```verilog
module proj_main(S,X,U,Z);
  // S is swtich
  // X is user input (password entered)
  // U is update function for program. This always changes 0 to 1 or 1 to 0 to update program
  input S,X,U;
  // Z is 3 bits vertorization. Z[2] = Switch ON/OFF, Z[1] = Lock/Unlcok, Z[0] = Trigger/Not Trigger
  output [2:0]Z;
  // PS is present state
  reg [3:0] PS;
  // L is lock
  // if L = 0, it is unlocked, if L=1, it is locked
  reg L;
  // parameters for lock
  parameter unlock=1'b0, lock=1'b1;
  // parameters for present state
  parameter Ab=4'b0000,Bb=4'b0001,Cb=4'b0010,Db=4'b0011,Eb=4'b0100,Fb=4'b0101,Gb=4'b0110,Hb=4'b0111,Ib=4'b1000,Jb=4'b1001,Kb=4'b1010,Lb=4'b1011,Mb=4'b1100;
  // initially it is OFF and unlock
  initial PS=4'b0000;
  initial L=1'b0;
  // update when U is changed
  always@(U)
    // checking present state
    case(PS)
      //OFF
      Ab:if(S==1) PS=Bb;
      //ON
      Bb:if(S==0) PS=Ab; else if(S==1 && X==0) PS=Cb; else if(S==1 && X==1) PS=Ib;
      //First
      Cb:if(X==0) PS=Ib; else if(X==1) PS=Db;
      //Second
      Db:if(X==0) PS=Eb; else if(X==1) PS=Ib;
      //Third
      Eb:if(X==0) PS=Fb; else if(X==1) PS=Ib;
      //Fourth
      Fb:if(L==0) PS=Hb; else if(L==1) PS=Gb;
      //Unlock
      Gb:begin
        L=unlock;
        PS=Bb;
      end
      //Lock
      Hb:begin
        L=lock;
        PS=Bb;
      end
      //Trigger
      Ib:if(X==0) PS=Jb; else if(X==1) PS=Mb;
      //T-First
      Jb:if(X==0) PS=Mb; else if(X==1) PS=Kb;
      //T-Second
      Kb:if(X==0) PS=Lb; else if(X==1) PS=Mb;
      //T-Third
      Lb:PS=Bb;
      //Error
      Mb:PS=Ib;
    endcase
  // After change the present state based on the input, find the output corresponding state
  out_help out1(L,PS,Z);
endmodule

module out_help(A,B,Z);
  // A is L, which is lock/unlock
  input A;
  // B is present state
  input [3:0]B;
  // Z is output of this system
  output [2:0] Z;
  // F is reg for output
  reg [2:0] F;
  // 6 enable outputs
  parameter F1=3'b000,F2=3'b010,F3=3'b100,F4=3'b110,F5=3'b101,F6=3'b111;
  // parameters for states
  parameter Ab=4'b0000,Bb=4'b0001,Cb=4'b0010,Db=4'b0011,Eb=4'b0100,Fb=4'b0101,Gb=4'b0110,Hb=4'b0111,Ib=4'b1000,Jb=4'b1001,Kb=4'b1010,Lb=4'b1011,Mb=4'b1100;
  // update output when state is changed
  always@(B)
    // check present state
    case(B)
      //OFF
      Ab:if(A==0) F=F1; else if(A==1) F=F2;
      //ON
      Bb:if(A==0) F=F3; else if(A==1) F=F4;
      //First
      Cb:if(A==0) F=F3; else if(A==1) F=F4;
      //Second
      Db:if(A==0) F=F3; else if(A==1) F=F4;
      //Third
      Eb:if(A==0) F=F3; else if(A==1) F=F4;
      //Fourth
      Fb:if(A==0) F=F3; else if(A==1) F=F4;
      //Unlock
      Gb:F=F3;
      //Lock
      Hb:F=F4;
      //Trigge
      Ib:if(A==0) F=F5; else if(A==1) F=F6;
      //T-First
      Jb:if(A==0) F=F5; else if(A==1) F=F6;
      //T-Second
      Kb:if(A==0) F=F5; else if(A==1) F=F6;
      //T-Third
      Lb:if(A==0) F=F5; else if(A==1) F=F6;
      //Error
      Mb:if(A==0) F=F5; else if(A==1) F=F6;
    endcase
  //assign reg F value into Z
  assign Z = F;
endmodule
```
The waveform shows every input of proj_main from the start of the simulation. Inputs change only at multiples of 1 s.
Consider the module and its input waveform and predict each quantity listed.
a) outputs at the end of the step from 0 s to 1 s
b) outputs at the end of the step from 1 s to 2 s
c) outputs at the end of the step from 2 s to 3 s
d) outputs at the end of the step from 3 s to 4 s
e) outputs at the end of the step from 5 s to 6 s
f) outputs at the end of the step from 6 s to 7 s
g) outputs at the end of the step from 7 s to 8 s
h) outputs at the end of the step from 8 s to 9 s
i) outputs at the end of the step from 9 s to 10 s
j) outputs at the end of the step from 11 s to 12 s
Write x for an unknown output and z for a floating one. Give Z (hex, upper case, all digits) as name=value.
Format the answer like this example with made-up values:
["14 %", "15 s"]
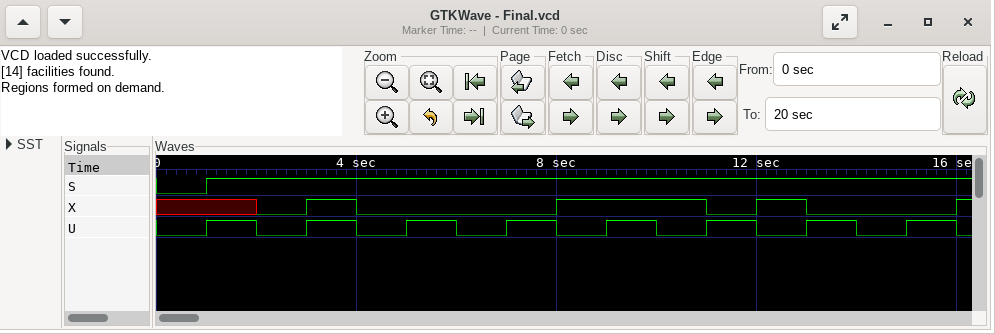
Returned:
["Z=0", "Z=4", "Z=4", "Z=4", "Z=4", "Z=6", "Z=6", "Z=7", "Z=7", "Z=7"]
